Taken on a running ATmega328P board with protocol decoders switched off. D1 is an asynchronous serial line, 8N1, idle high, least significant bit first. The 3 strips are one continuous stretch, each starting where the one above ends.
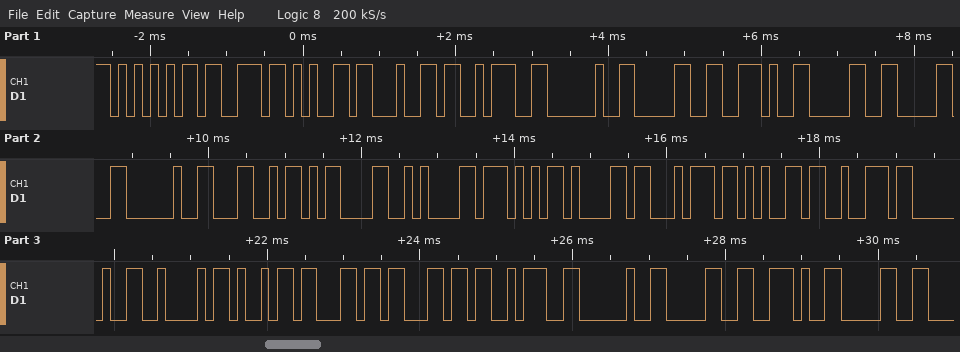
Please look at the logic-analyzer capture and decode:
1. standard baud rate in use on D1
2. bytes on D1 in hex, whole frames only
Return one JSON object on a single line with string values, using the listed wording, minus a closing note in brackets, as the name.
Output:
{"standard baud rate in use on D1": "9600 baud", "bytes on D1 in hex, whole frames only": "55 73 65 64 3A 20 30 2E 30 30 20 4C 0D 0A 57 61 74 65 72 20 42 69 6C 6C 3A 20 30 2E 30"}
